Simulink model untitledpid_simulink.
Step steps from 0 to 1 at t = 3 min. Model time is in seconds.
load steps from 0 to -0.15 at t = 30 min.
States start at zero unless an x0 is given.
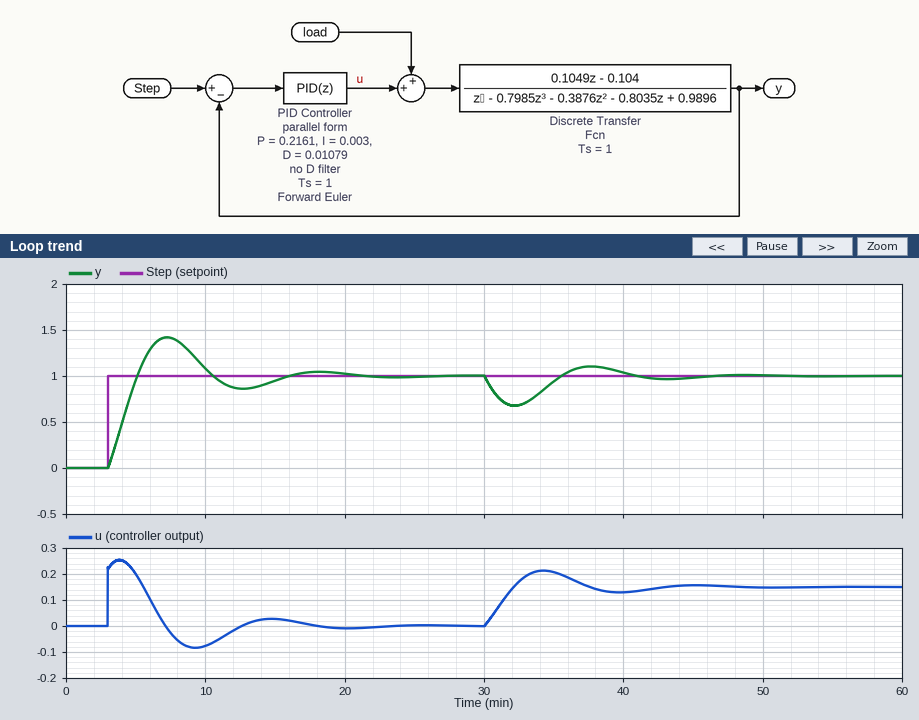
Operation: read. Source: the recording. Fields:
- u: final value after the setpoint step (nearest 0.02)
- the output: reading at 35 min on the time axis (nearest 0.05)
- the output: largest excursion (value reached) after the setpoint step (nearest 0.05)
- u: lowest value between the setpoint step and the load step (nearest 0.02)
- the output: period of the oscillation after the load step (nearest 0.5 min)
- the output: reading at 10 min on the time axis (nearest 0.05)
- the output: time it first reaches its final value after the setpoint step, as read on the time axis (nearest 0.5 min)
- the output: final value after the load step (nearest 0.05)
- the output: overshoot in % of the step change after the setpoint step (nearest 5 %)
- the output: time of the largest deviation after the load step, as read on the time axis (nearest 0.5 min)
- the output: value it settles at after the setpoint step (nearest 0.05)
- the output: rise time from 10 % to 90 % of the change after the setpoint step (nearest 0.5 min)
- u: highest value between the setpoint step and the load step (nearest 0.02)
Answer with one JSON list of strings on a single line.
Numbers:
["0.00", "0.95", "1.40", "-0.08", "11.0 min", "1.10", "5.0 min", "1.00", "40 %", "32.0 min", "1.00", "1.5 min", "0.26"]
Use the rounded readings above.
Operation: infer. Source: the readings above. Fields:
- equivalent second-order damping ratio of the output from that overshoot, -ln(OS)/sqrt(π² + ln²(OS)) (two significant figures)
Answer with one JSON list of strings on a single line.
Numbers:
["0.28"]
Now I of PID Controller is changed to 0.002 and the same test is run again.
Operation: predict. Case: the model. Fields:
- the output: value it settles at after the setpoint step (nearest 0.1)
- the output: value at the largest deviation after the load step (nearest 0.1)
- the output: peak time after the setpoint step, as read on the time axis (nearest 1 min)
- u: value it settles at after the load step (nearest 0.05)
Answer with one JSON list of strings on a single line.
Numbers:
["1.0", "0.6", "8 min", "0.15"]
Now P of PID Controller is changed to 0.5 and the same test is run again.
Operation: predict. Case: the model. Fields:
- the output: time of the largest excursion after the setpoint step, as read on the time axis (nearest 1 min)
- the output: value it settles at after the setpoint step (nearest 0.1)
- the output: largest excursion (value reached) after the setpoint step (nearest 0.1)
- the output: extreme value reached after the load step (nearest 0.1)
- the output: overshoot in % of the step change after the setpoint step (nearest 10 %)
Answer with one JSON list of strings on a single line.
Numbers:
["6 min", "1.0", "1.2", "0.8", "20 %"]
